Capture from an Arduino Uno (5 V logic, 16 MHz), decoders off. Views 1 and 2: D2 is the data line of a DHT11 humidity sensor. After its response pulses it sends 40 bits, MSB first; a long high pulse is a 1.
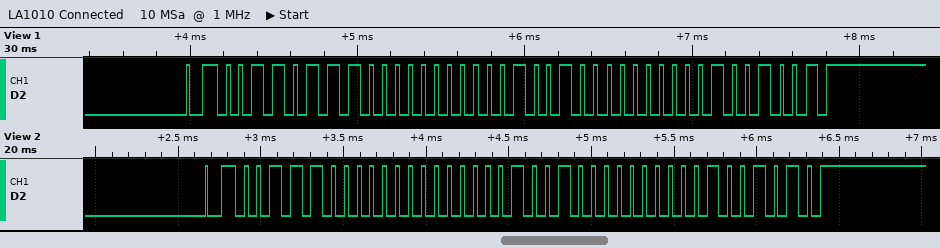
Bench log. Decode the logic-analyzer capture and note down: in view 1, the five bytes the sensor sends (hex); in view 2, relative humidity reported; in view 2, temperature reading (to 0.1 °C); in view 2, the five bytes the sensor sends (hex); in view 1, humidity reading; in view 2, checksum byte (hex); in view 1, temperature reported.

37 00 12 00 49
56 %
18.0 °C
38 00 12 00 4A
55 %
0x4A
18.0 °C
